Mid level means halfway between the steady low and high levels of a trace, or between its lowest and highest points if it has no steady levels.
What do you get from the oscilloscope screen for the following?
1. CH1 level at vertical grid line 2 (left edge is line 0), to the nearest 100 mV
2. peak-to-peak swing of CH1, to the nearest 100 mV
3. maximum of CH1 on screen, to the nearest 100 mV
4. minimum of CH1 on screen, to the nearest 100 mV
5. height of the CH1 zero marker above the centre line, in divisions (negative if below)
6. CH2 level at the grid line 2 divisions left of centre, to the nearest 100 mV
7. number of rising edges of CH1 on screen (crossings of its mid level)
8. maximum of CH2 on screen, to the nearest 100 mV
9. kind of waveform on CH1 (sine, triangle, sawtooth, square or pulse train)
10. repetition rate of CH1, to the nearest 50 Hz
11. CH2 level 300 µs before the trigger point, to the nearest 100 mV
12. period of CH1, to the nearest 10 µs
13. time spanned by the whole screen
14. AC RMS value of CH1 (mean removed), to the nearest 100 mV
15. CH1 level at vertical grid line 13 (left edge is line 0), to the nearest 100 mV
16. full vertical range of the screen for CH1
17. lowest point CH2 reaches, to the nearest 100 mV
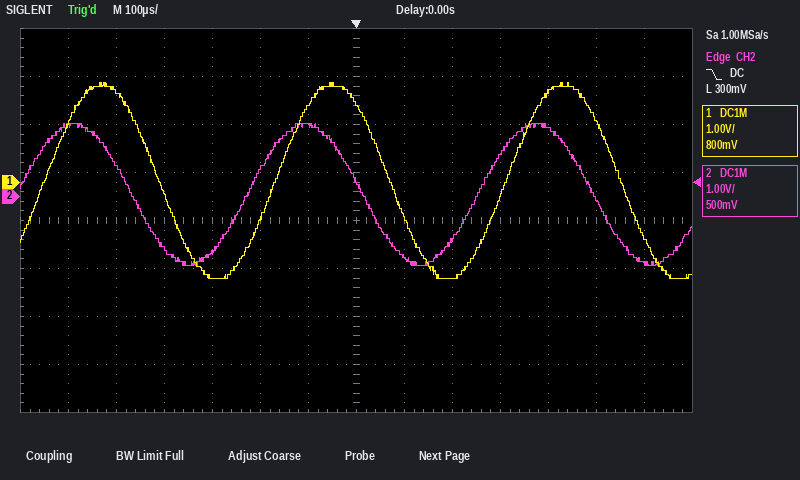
1.9 V
4.1 V
2.1 V
-2.0 V
+0.8 div
600 mV
3
1.5 V
sine
2.10 kHz
-1.2 V
480 µs
1.4 ms
1.4 V
-1.1 V
8 V
-1.4 V
